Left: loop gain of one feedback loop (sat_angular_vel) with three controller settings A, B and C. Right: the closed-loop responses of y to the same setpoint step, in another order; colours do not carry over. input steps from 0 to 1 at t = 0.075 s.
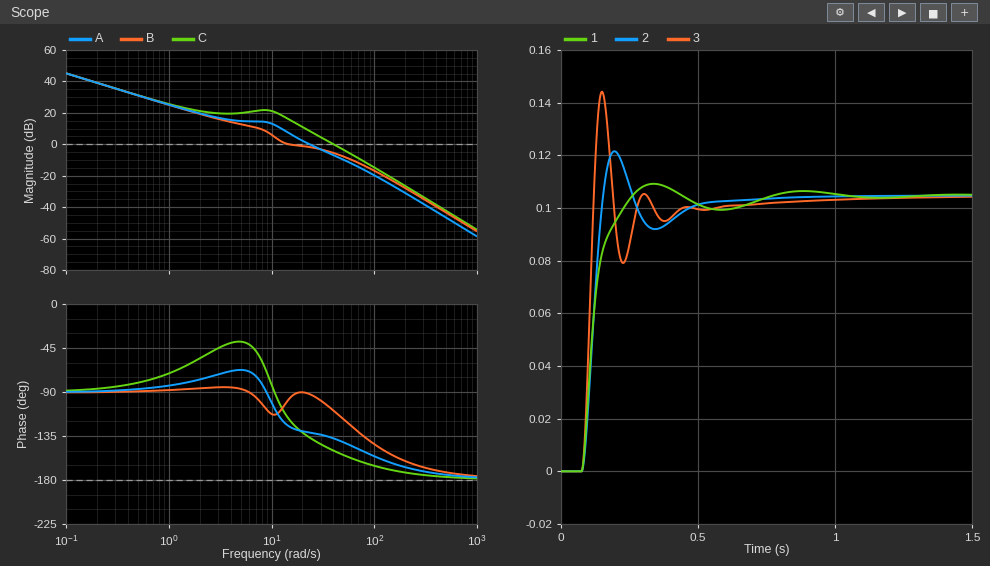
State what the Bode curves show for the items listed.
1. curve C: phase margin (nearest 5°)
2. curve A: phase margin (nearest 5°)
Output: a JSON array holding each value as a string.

["30°", "50°"]
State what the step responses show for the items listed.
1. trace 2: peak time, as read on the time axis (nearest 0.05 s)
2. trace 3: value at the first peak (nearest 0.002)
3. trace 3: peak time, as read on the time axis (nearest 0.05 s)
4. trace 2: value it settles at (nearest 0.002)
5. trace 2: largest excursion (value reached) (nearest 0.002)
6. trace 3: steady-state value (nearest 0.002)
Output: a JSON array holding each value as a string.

["0.20 s", "0.144", "0.15 s", "0.104", "0.122", "0.104"]
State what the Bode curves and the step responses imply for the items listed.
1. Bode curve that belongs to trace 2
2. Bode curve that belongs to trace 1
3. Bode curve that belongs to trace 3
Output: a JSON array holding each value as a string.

["A", "B", "C"]
